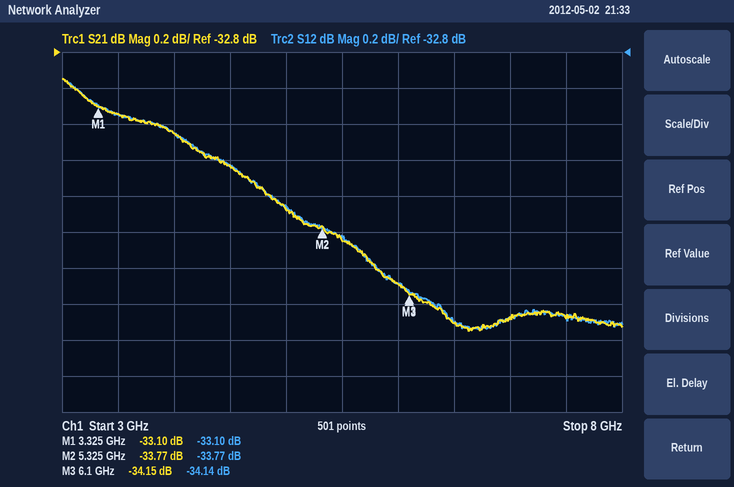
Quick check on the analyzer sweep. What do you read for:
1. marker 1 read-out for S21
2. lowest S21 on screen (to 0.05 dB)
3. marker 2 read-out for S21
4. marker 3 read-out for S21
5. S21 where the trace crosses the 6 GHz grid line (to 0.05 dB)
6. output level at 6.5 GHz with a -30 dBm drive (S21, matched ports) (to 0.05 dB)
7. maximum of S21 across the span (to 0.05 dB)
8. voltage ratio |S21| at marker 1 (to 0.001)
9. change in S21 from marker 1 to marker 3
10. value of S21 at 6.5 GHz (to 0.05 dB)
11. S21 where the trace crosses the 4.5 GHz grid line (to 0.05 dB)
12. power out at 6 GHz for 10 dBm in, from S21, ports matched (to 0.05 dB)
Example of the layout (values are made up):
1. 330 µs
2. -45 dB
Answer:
1. -33.10 dB
2. -34.35 dB
3. -33.77 dB
4. -34.15 dB
5. -34.10 dB
6. -64.30 dBm
7. -32.95 dB
8. 0.022
9. -1.05 dB
10. -34.30 dB
11. -33.45 dB
12. -24.10 dBm
